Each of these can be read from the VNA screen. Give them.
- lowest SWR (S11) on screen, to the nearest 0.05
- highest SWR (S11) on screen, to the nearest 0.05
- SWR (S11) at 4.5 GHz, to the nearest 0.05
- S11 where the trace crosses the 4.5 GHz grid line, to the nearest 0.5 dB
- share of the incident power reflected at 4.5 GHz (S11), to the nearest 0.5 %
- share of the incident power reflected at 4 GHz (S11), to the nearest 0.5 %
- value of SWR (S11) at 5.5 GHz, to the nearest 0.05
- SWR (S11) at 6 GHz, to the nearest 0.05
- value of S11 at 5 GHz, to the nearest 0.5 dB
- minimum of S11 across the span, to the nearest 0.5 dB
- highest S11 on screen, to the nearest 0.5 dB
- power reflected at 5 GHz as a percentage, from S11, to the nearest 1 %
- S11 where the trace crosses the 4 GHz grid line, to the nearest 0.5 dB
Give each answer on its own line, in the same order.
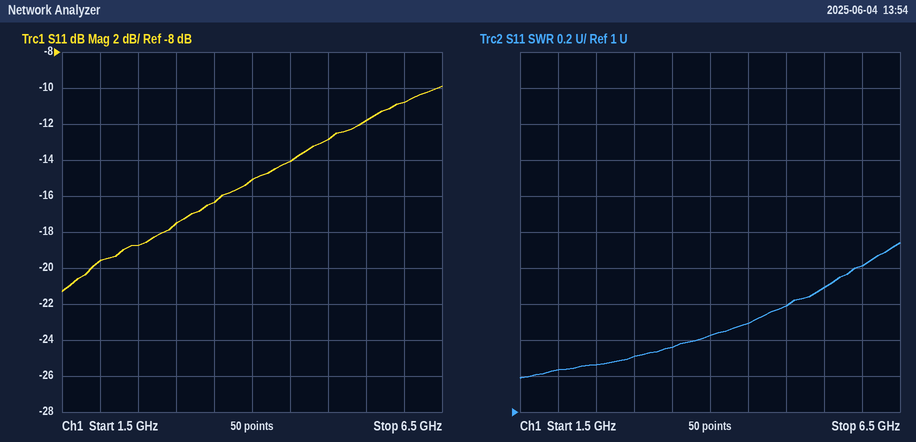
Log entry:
1.20
1.95
1.50
-14.0 dB
4.0 %
3.0 %
1.70
1.80
-13.0 dB
-21.5 dB
-10.0 dB
5 %
-15.0 dB
